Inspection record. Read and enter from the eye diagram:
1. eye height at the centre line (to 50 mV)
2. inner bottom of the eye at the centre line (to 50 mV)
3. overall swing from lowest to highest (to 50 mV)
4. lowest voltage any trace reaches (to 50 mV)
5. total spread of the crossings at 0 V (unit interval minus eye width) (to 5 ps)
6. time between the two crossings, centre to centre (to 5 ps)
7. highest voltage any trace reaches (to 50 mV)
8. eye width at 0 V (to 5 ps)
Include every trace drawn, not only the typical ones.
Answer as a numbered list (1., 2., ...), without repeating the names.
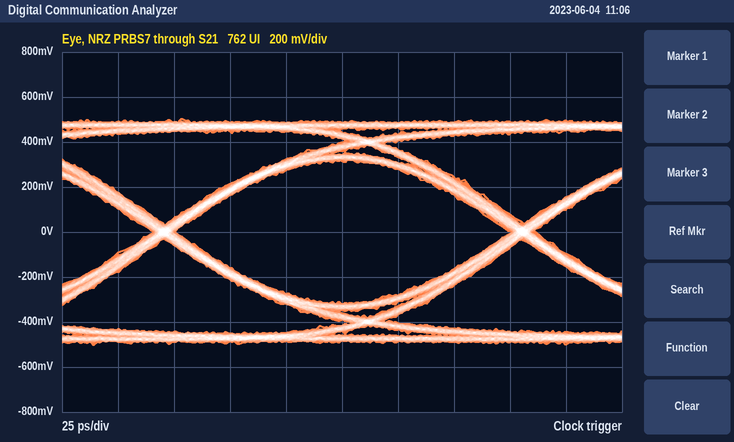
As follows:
1. 650 mV
2. -300 mV
3. 1.00 V
4. -500 mV
5. 10 ps
6. 160 ps
7. 500 mV
8. 150 ps
